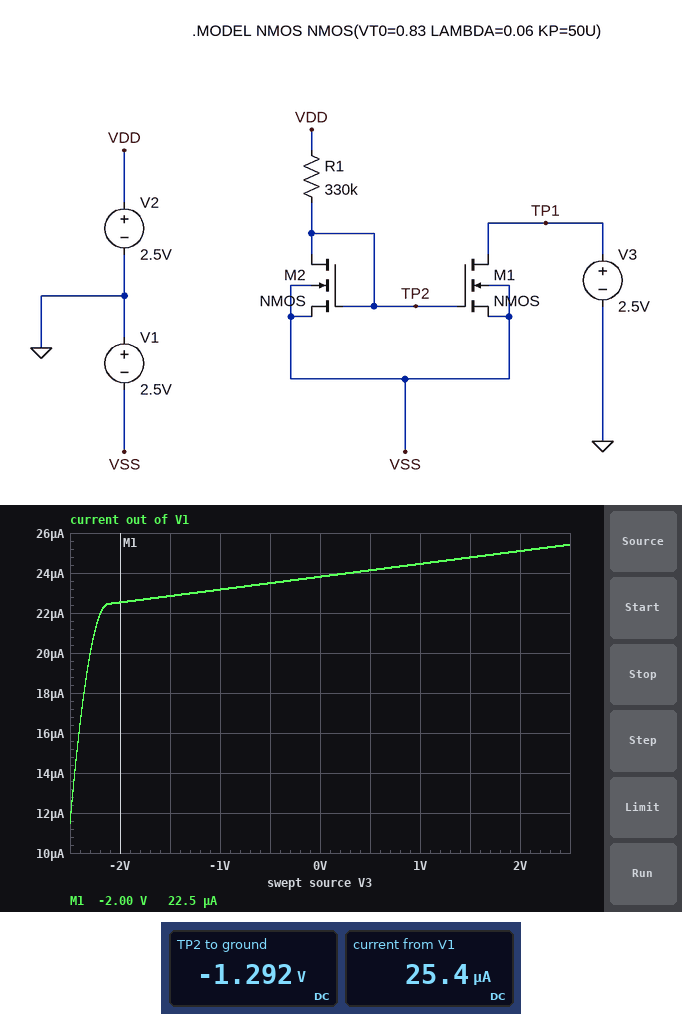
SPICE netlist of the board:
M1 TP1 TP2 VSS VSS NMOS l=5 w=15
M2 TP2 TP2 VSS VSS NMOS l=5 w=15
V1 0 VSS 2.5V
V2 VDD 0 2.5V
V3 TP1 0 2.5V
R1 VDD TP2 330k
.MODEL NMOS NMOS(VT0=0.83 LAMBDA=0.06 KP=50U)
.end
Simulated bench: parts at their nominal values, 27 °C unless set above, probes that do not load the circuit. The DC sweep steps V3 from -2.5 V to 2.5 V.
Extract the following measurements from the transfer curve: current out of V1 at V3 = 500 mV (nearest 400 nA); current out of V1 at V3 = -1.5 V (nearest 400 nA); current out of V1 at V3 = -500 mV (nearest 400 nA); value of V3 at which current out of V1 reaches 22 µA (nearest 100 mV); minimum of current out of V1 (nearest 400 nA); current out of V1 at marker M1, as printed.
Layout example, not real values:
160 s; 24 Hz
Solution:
24.0 µA; 22.8 µA; 23.6 µA; -2.2 V; 11.6 µA; 22.5 µA
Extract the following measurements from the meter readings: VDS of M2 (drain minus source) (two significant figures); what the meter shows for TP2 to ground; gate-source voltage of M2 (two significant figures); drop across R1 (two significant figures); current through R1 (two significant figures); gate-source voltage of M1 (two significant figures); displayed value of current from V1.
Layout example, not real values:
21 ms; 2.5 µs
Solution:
1.2 V; -1.292 V; 1.2 V; 3.8 V; 11 µA; 1.2 V; 25.4 µA
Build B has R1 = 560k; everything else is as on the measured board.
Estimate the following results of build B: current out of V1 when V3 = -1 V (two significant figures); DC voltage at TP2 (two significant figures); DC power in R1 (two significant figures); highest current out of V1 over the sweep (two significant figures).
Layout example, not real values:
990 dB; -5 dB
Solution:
14 µA; -1.4 V; 27 µW; 15 µA
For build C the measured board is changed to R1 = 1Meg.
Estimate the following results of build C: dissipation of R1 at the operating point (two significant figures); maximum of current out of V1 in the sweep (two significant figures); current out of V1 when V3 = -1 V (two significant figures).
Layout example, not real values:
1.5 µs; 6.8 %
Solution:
16 µW; 8.8 µA; 8.0 µA
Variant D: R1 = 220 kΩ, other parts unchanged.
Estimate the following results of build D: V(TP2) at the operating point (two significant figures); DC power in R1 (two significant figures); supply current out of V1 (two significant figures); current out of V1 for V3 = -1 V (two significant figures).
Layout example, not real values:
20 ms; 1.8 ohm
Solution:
-1.2 V; 63 µW; 37 µA; 34 µA
